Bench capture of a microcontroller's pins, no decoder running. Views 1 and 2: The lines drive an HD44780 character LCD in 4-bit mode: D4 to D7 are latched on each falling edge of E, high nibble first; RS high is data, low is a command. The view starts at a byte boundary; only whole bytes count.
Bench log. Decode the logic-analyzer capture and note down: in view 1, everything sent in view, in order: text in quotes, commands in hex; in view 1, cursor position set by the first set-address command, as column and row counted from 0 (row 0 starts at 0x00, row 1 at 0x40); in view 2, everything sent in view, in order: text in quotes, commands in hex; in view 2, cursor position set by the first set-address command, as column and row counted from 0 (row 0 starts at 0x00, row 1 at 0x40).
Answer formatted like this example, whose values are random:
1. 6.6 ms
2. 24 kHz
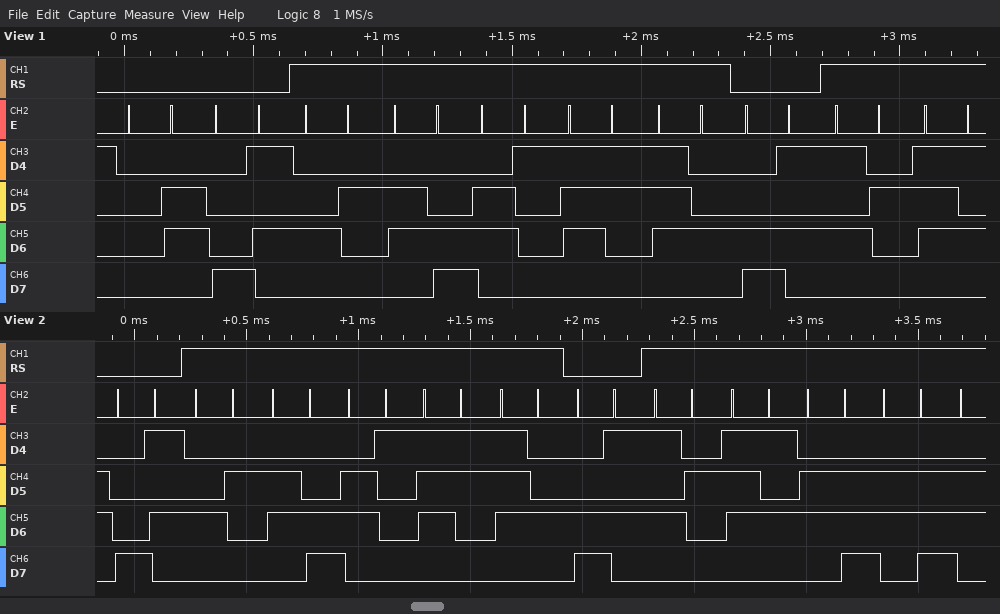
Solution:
1. 0x06 0x85 "Blast" 0xC5 "Ru"
2. column 5, row 0
3. 0x85 "Blast" 0xC5 "Runn"
4. column 5, row 0
